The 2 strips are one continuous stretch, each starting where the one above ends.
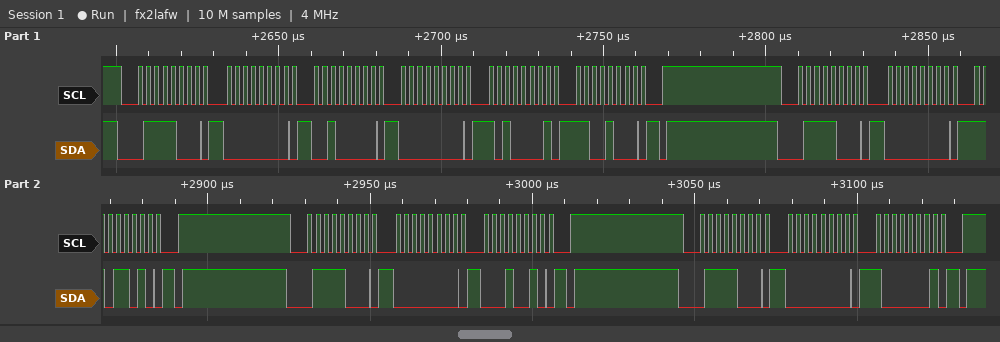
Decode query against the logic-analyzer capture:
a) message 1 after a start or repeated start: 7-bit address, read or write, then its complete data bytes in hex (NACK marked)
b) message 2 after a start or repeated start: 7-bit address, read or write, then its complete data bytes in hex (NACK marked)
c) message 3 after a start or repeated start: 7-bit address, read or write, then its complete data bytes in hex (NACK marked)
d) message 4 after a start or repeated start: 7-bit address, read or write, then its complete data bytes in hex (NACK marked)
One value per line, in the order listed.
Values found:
0x3C write: 00 20 00 A1 C8
0x3C write: 00 DA
0x3C write: 00 12
0x3C write: 00 81
